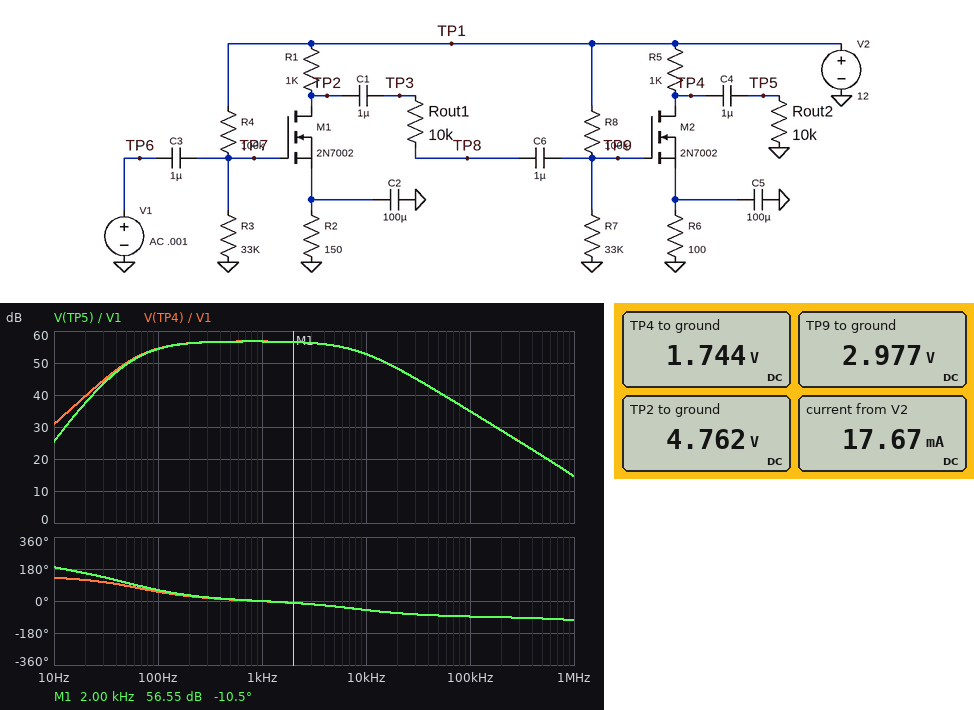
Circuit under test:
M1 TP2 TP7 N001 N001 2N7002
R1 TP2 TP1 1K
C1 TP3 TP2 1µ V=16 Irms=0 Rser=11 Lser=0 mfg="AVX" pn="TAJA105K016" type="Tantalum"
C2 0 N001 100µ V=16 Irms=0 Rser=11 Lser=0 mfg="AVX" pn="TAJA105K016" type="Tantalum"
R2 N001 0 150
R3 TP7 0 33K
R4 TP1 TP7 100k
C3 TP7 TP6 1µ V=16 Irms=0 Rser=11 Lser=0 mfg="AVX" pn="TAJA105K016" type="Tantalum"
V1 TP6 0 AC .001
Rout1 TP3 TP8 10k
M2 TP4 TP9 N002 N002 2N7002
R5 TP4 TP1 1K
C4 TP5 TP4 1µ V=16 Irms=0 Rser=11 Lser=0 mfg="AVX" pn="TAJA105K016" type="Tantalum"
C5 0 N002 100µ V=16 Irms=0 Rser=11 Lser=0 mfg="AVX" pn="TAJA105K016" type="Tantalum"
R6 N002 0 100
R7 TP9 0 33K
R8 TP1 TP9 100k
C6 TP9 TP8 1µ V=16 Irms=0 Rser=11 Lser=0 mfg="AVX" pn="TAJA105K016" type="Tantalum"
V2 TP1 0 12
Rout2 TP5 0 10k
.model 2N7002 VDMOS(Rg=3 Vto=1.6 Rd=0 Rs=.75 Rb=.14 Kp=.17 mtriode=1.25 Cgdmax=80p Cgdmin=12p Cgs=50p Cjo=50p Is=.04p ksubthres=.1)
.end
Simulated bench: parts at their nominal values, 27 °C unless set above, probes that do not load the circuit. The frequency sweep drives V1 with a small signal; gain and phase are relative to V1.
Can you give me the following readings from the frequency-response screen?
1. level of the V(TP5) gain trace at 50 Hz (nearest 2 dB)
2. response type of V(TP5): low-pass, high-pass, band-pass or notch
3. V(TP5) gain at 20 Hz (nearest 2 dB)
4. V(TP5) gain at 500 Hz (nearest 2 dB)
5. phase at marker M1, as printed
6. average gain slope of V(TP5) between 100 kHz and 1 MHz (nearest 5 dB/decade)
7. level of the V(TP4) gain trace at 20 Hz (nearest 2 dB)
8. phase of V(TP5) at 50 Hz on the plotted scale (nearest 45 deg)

50 dB
band-pass
38 dB
56 dB
-10.5 deg
-20 dB/decade
40 dB
90 deg
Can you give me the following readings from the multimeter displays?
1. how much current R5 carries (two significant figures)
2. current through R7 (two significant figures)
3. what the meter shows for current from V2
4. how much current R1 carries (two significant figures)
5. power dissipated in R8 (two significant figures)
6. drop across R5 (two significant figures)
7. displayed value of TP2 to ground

10 mA
90 µA
17.67 mA
7.2 mA
810 µW
10 V
4.762 V
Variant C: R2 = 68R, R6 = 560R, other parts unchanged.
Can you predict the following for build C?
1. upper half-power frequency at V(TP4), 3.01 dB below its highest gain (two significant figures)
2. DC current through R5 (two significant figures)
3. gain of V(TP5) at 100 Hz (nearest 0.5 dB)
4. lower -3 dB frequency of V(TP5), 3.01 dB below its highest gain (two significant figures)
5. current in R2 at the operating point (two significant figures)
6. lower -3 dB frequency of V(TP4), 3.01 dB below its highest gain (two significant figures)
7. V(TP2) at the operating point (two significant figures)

72 kHz
2.2 mA
6.0 dB
39 Hz
11 mA
33 Hz
860 mV
